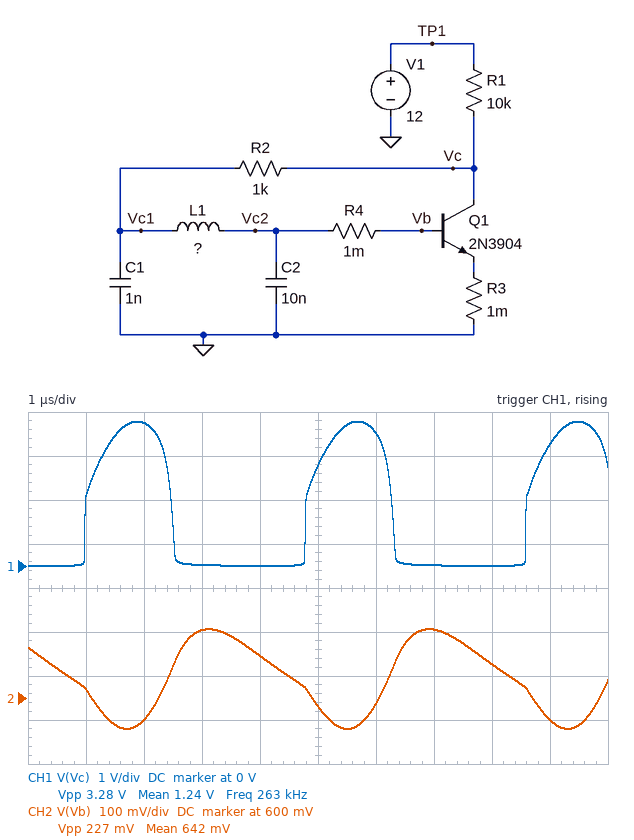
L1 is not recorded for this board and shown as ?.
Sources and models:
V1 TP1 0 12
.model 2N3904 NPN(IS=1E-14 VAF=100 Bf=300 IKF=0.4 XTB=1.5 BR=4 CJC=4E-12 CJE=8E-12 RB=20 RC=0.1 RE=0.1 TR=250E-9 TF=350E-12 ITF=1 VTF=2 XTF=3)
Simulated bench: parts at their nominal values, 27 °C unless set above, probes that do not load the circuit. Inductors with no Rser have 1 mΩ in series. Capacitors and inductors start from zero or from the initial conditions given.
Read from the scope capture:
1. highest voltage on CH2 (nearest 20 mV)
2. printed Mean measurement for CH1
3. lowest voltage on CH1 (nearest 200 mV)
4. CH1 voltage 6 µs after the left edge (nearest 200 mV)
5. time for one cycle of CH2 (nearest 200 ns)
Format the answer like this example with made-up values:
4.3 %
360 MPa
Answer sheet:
760 mV
1.24 V
0 V
3.0 V
3.8 µs
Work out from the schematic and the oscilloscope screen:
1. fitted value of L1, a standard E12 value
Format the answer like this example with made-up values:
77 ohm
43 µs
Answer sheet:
390 µH
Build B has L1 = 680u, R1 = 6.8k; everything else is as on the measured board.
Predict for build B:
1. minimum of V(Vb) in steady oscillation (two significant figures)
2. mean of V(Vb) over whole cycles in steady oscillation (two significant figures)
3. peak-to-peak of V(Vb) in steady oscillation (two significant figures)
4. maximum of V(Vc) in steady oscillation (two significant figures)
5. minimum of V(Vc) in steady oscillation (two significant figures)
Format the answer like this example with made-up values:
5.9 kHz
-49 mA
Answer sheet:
550 mV
670 mV
220 mV
4.0 V
6.0 mV
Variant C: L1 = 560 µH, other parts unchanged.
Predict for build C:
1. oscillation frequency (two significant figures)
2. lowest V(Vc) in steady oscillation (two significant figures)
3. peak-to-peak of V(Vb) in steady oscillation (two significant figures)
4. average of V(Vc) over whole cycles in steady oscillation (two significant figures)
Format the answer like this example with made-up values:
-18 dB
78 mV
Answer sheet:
220 kHz
4.2 mV
210 mV
1.1 V
